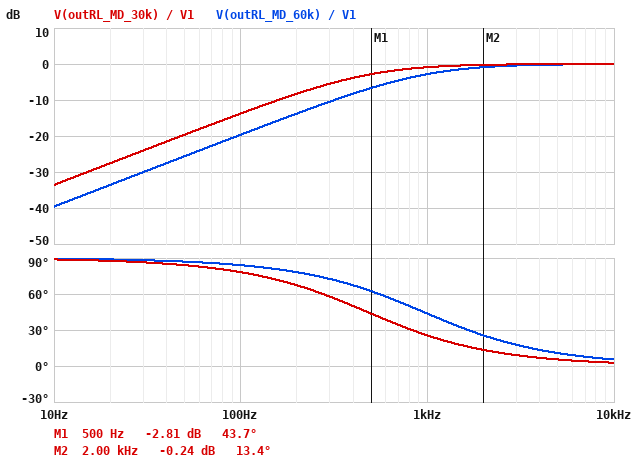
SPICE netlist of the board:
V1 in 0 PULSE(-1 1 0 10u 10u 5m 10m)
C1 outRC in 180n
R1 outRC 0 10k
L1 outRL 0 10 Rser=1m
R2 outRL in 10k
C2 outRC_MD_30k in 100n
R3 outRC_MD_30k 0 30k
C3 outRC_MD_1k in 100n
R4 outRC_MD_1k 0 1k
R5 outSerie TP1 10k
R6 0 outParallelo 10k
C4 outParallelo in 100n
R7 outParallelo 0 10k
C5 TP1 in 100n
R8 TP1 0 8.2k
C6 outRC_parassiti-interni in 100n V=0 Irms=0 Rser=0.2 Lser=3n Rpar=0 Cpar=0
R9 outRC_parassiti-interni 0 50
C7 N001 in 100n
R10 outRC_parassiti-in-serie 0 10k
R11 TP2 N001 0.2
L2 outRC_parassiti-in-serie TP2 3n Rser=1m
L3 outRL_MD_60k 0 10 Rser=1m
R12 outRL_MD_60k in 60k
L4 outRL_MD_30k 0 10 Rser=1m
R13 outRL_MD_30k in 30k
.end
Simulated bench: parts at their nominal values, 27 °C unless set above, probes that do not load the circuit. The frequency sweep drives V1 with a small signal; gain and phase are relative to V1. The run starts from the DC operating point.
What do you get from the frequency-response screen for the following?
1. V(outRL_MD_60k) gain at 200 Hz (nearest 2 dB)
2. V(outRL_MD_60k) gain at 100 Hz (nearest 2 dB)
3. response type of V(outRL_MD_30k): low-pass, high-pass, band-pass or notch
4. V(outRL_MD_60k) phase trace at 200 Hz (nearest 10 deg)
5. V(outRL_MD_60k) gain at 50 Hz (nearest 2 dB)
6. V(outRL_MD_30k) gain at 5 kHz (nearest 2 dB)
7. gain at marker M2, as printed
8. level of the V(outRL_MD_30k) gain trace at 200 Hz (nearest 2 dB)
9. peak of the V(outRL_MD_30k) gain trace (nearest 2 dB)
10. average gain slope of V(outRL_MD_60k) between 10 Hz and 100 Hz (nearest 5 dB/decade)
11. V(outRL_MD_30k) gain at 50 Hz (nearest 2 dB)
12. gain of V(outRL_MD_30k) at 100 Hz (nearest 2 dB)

-14 dB
-20 dB
high-pass
80 deg
-26 dB
0 dB
-0.24 dB
-8 dB
0 dB
20 dB/decade
-20 dB
-14 dB
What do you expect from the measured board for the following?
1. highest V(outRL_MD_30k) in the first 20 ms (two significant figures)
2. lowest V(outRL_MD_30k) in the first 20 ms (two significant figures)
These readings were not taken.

2.0 V
-2.0 V
